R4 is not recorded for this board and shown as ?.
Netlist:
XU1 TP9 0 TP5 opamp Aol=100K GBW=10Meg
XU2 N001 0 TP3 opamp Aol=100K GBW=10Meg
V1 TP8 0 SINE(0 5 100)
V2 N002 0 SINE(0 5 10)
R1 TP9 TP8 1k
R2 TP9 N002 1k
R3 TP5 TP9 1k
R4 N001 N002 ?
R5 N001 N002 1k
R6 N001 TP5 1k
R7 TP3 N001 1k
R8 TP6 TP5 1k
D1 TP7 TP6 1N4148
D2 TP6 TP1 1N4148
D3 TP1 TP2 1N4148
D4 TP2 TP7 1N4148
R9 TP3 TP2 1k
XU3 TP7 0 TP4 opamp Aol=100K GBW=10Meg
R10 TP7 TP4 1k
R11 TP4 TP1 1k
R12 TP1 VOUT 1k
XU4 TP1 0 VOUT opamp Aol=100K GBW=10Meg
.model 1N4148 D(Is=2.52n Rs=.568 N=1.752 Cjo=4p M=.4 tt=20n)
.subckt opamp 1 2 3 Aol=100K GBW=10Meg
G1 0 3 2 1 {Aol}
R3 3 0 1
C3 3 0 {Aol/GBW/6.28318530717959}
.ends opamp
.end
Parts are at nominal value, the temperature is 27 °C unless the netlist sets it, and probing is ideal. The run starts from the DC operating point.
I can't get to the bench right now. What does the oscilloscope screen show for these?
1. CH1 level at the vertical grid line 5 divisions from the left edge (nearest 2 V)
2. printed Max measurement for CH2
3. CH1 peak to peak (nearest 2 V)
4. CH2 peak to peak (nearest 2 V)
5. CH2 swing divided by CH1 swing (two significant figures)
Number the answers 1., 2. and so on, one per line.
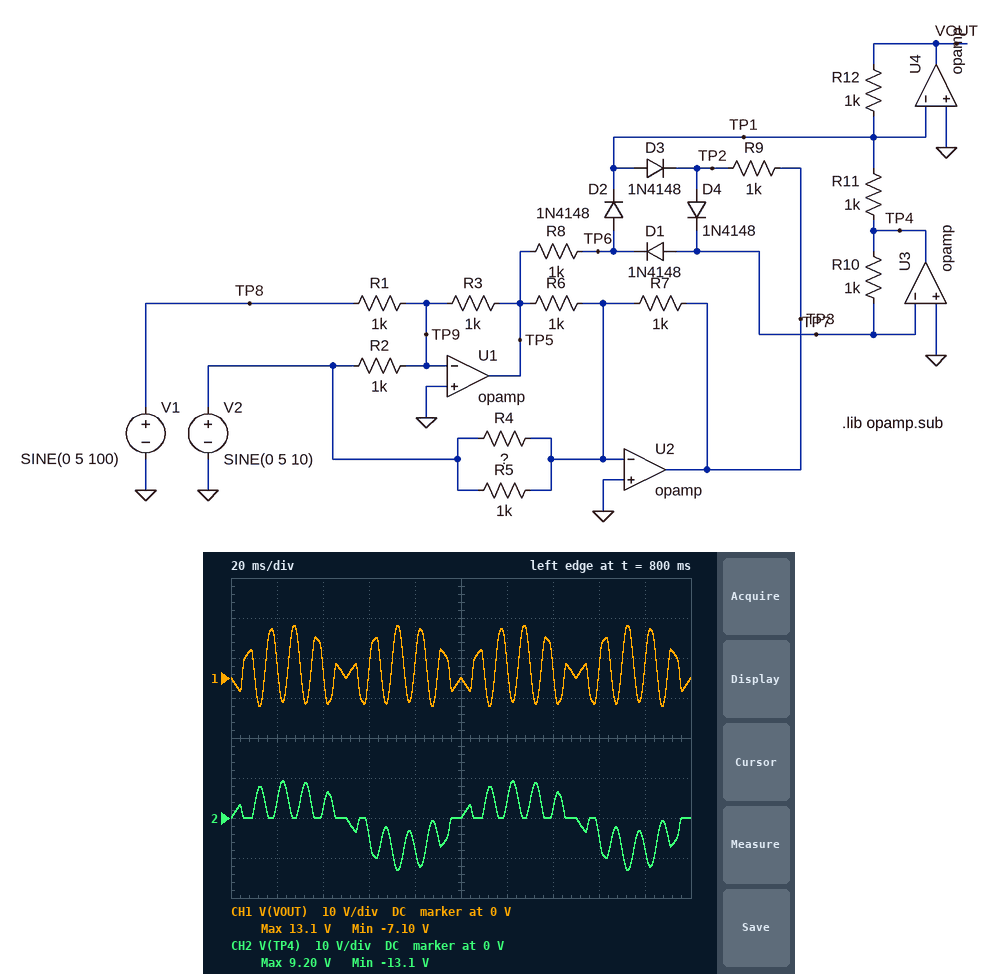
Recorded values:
1. 0 V
2. 9.20 V
3. 20 V
4. 22 V
5. 1.1
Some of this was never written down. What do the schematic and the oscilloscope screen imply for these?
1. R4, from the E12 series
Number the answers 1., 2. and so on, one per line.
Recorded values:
1. 560 Ω
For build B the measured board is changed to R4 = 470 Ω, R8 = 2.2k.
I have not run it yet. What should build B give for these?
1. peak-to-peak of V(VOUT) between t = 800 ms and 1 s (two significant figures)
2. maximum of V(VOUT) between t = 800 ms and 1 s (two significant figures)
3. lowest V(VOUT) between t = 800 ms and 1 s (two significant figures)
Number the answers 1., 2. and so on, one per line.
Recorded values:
1. 18 V
2. 15 V
3. -3.0 V
